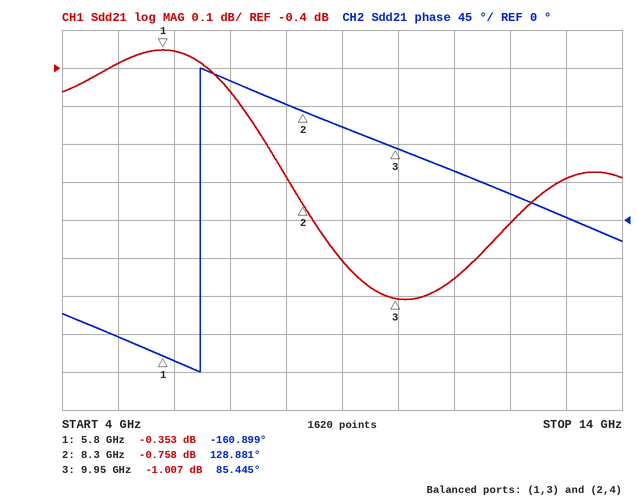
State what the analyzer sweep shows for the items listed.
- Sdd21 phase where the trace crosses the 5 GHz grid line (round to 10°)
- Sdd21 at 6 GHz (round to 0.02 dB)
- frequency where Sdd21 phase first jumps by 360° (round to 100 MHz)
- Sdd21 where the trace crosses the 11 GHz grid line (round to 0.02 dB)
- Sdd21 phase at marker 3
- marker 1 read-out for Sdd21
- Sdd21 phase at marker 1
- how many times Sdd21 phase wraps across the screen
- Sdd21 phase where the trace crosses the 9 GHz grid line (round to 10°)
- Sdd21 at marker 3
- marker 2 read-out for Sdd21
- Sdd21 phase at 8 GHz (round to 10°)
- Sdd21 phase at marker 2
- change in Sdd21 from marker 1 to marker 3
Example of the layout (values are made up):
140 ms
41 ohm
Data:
-140°
-0.36 dB
6.5 GHz
-0.96 dB
85.445°
-0.353 dB
-160.899°
1
110°
-1.007 dB
-0.758 dB
140°
128.881°
-0.654 dB
